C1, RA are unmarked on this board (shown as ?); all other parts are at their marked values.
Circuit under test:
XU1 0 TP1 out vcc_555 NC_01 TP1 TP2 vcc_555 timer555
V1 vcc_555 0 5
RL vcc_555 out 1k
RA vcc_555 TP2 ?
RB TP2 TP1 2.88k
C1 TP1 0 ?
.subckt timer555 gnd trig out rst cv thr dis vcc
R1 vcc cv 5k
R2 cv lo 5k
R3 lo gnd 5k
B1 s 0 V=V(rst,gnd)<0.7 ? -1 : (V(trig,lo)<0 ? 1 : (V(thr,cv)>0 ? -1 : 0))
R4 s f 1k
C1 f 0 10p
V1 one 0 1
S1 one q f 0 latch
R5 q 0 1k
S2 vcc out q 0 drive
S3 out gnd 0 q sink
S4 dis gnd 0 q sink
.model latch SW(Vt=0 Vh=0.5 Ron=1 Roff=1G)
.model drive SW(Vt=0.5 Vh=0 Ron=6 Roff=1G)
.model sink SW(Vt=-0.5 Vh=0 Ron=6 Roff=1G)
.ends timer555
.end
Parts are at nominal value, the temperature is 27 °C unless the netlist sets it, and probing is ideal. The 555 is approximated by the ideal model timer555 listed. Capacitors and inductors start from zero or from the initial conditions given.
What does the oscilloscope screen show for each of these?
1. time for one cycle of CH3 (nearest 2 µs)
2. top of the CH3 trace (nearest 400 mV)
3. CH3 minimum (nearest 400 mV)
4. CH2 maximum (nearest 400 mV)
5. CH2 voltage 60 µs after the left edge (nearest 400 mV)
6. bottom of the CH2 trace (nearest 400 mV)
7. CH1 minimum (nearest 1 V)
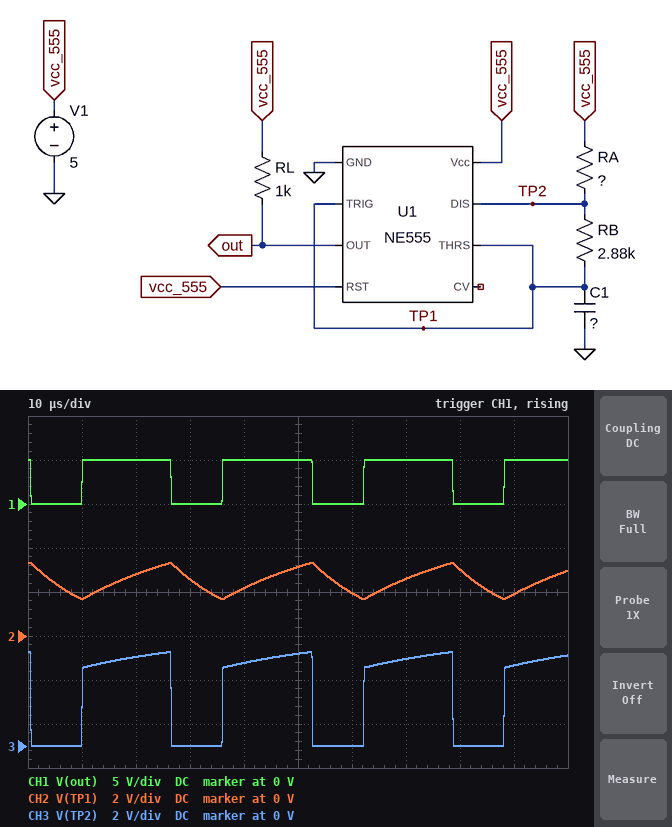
26 µs
4.4 V
0 V
3.2 V
2.0 V
1.6 V
0 V
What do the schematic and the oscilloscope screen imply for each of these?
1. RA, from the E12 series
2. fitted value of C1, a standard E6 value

2.2 kΩ
4.7 nF
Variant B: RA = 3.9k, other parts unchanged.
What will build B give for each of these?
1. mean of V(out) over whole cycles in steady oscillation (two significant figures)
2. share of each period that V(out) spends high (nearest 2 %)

3.5 V
70 %
